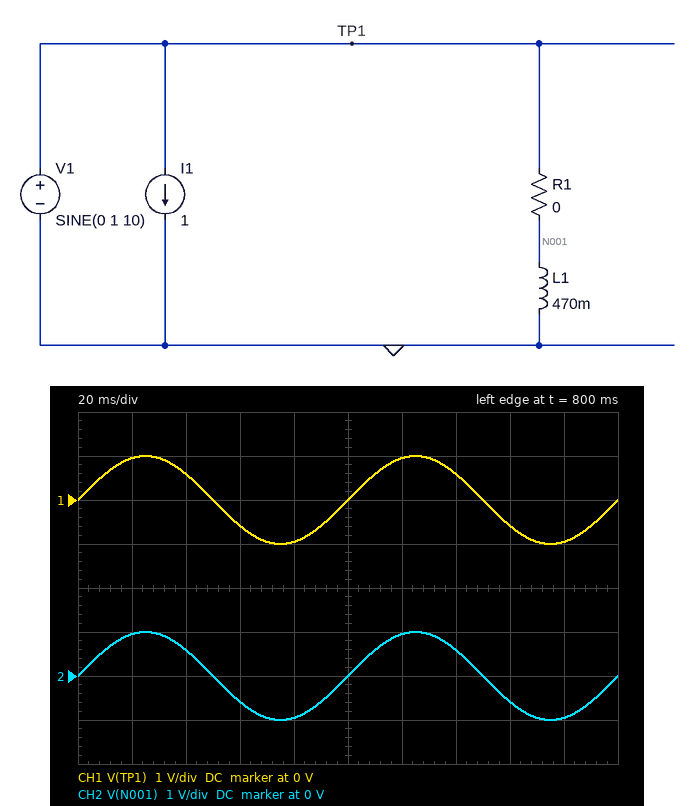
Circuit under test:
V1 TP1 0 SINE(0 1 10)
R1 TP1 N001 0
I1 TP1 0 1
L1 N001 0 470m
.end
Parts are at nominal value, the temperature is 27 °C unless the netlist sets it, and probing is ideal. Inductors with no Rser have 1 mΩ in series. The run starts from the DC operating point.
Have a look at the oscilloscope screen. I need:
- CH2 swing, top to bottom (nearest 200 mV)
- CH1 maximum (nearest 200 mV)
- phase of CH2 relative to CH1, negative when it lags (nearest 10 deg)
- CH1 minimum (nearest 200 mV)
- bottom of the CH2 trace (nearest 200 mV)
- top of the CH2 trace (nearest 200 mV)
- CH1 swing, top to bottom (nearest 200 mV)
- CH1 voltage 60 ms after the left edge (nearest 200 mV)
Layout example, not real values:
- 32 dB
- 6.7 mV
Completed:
- 2.0 V
- 1.0 V
- 0 deg
- -1.0 V
- -1.0 V
- 1.0 V
- 2.0 V
- -600 mV
